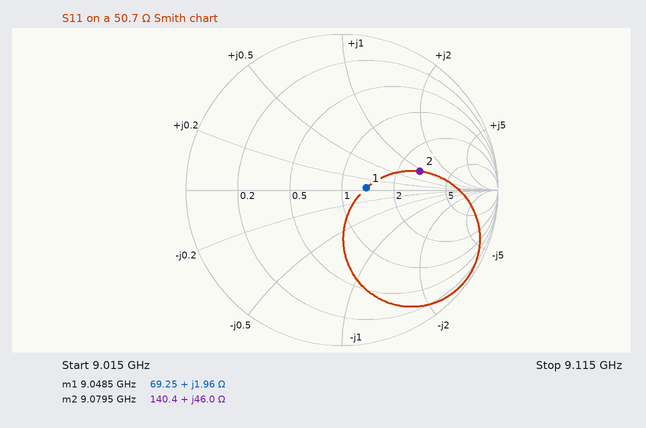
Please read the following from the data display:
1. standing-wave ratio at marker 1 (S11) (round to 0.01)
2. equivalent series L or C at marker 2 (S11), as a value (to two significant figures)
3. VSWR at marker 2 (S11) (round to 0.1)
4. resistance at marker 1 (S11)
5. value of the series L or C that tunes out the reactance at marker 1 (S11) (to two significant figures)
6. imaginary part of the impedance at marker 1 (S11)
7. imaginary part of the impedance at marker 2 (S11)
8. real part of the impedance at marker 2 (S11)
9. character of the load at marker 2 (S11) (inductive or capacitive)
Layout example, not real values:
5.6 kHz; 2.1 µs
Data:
1.37; 810 pH; 3.1; 69.25 Ω; 9.0 pF; +1.96 Ω; +46.0 Ω; 140.4 Ω; inductive
